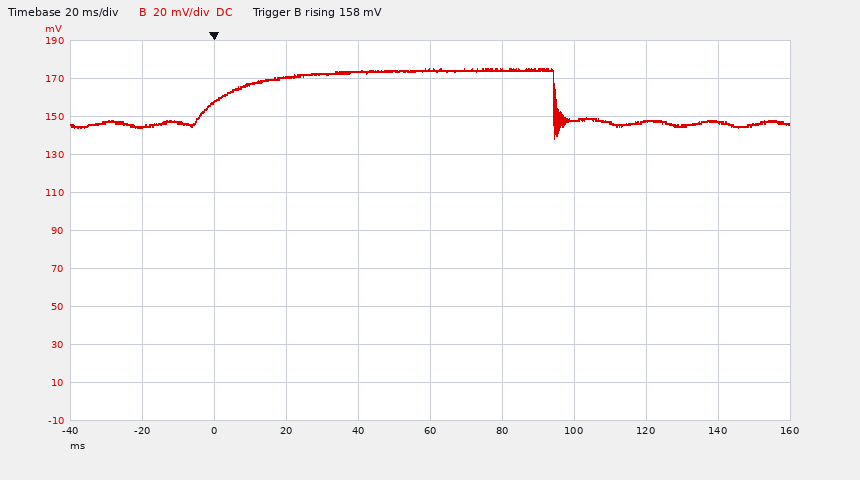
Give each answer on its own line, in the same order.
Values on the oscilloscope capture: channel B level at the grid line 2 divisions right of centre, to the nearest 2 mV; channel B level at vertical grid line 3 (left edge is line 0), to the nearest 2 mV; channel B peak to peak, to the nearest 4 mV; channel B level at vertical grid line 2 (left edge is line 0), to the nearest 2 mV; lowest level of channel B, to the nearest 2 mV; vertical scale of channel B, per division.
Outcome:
148 mV
170 mV
36 mV
158 mV
138 mV
20 mV
